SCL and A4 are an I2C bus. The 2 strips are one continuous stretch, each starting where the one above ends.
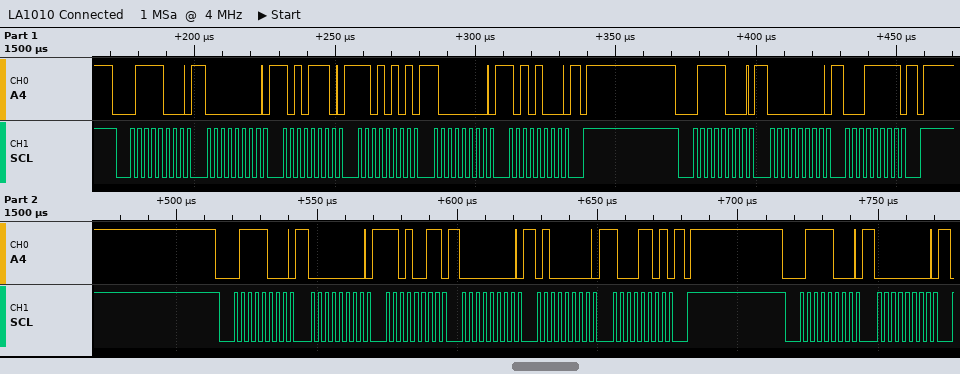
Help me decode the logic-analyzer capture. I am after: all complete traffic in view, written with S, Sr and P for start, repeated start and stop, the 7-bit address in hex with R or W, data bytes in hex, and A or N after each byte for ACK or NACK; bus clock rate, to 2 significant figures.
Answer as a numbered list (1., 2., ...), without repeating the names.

1. S 3CW A 00 A AE A D5 A 80 A A8 A P S 3CW A 00 A 1F A P S 3CW A 00 A D3 A 00 A 40 A 8D A P S 3CW A 00 A
2. 400 kHz
